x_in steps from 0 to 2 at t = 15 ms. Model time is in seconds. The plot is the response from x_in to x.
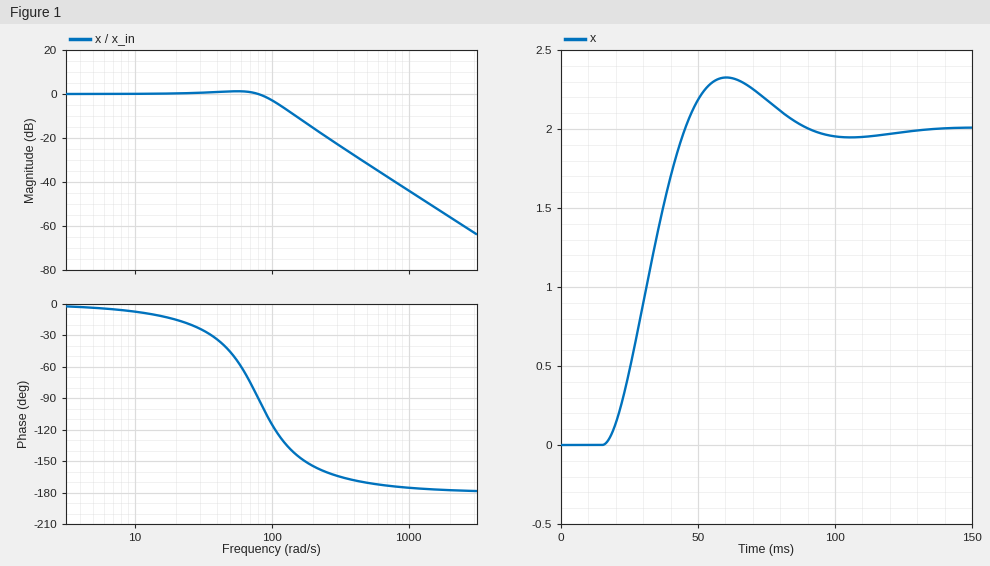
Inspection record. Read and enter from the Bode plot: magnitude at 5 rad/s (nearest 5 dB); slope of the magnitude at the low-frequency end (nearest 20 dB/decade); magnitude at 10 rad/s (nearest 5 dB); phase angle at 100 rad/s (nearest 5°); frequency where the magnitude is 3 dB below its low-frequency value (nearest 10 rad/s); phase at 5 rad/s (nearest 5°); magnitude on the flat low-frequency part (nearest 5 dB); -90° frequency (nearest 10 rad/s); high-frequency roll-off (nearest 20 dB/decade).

0 dB
0 dB/decade
0 dB
-115°
100 rad/s
-5°
0 dB
80 rad/s
-40 dB/decade
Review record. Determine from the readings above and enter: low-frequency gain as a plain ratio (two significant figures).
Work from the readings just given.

1.0
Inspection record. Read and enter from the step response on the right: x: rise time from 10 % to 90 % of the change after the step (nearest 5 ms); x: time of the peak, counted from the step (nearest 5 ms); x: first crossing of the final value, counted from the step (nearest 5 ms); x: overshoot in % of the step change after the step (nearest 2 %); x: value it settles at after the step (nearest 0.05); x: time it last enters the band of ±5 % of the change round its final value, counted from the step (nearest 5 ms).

20 ms
45 ms
30 ms
16 %
2.00
65 ms
